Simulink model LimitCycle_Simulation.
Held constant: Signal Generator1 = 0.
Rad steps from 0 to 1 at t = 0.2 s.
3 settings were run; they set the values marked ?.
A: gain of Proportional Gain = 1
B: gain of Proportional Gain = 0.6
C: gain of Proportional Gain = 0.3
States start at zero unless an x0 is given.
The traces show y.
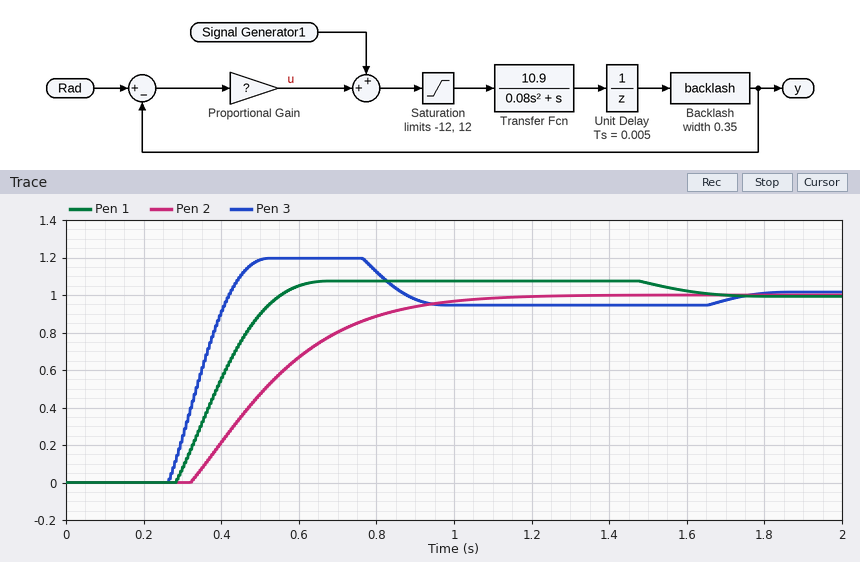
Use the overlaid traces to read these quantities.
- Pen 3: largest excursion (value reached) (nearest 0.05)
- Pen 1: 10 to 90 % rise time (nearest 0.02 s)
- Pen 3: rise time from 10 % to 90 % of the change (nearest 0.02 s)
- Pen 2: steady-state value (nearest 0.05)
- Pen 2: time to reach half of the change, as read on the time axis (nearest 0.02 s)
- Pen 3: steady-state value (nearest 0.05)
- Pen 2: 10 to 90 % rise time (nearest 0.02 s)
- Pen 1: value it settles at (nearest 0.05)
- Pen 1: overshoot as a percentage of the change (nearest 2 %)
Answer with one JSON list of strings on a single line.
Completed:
["1.20", "0.20 s", "0.12 s", "1.00", "0.52 s", "1.00", "0.46 s", "1.00", "8 %"]
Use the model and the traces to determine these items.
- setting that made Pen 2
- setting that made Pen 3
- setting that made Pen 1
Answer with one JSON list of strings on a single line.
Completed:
["C", "A", "B"]
